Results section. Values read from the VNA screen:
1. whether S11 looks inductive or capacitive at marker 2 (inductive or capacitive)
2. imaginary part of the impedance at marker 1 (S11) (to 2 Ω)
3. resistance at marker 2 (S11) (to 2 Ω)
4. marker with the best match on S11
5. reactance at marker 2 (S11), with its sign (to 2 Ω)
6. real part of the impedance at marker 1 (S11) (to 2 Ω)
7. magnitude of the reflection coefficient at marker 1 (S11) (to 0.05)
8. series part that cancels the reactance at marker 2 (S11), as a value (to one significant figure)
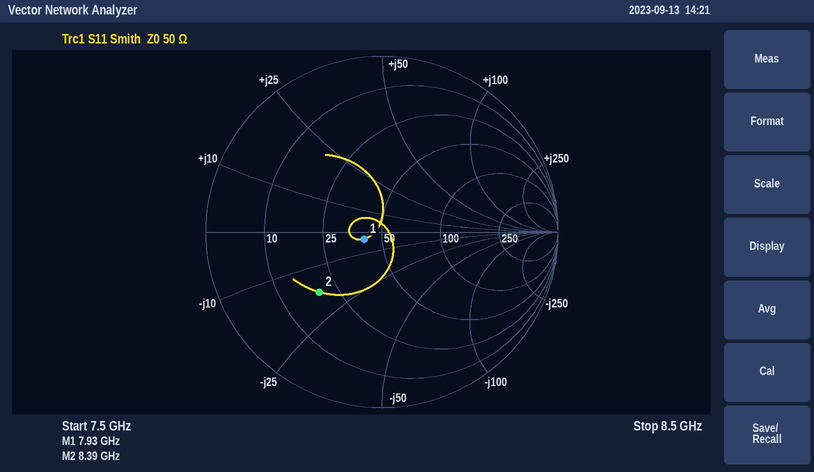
capacitive
-4 Ω
20 Ω
marker 1
-18 Ω
40 Ω
0.10
300 pH
